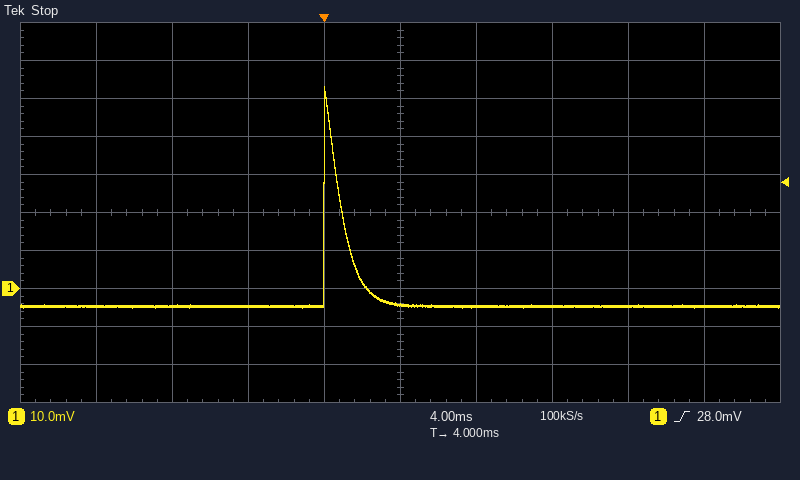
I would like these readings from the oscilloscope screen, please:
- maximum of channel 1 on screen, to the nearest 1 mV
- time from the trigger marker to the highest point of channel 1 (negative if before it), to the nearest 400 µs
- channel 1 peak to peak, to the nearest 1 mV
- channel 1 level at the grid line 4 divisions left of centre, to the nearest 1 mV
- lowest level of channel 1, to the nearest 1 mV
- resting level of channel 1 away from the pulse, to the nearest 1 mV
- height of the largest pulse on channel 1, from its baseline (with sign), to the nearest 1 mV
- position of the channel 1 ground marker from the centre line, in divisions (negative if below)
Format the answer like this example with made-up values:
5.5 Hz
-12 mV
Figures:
53 mV
0.0 ms
58 mV
-5 mV
-5 mV
-5 mV
+58 mV
-2.0 div
